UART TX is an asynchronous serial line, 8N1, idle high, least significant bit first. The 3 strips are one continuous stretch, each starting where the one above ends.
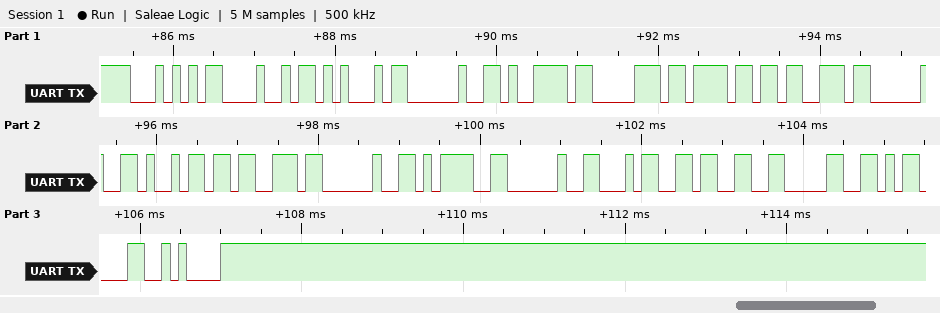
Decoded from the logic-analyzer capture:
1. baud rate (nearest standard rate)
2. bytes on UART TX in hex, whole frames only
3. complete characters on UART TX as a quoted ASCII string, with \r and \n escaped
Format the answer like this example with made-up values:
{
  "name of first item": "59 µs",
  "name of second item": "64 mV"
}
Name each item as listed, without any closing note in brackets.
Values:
{
  "baud rate": "9600 baud",
  "bytes on UART TX in hex, whole frames only": "54 48 45 20 79 70 6F 73 20 69 73 20 3D 20 34 33 30 0D 0A",
  "complete characters on UART TX as a quoted ASCII string, with \\r and \\n escaped": "\"THE ypos is = 430\\r\\n\""
}
